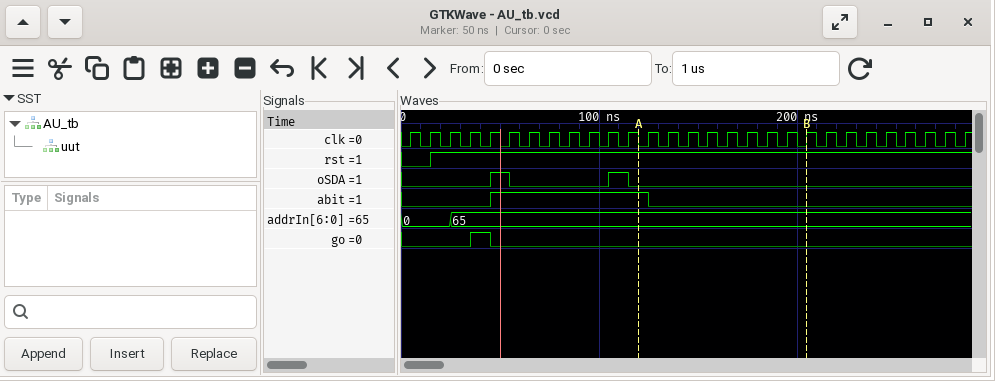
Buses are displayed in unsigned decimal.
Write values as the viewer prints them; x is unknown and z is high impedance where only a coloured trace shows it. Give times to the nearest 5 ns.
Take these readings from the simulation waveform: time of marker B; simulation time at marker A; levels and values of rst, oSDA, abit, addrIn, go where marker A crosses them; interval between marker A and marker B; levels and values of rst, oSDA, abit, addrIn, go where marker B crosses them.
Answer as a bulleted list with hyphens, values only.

- 205 ns
- 120 ns
- rst=1, oSDA=0, abit=1, addrIn=65, go=0
- 85 ns
- rst=1, oSDA=0, abit=0, addrIn=65, go=0
